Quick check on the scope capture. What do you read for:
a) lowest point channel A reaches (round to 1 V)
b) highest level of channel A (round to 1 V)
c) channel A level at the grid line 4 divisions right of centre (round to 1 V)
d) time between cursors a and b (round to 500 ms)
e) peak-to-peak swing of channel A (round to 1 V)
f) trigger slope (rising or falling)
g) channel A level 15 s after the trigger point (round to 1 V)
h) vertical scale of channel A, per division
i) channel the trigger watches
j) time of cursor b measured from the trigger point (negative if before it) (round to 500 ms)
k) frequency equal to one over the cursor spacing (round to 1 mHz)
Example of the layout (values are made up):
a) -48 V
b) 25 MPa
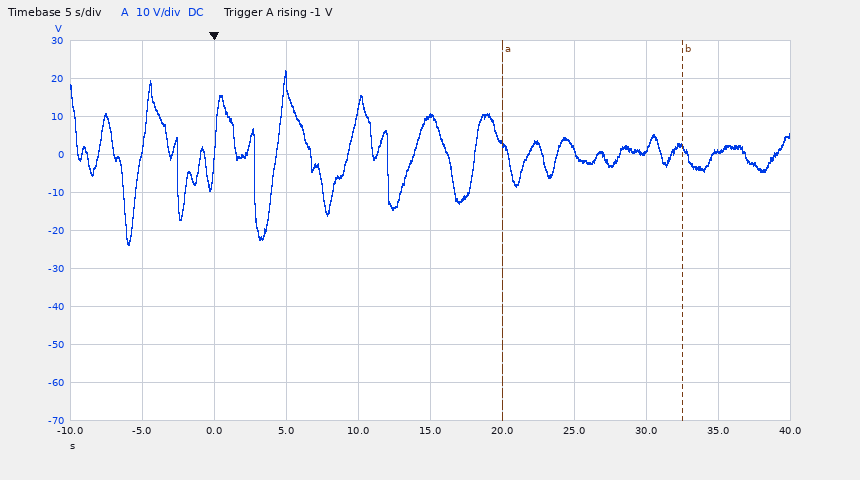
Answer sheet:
a) -24 V
b) 22 V
c) 1 V
d) 12.5 s
e) 46 V
f) rising
g) 10 V
h) 10 V
i) channel A
j) +32.5 s
k) 80 mHz
